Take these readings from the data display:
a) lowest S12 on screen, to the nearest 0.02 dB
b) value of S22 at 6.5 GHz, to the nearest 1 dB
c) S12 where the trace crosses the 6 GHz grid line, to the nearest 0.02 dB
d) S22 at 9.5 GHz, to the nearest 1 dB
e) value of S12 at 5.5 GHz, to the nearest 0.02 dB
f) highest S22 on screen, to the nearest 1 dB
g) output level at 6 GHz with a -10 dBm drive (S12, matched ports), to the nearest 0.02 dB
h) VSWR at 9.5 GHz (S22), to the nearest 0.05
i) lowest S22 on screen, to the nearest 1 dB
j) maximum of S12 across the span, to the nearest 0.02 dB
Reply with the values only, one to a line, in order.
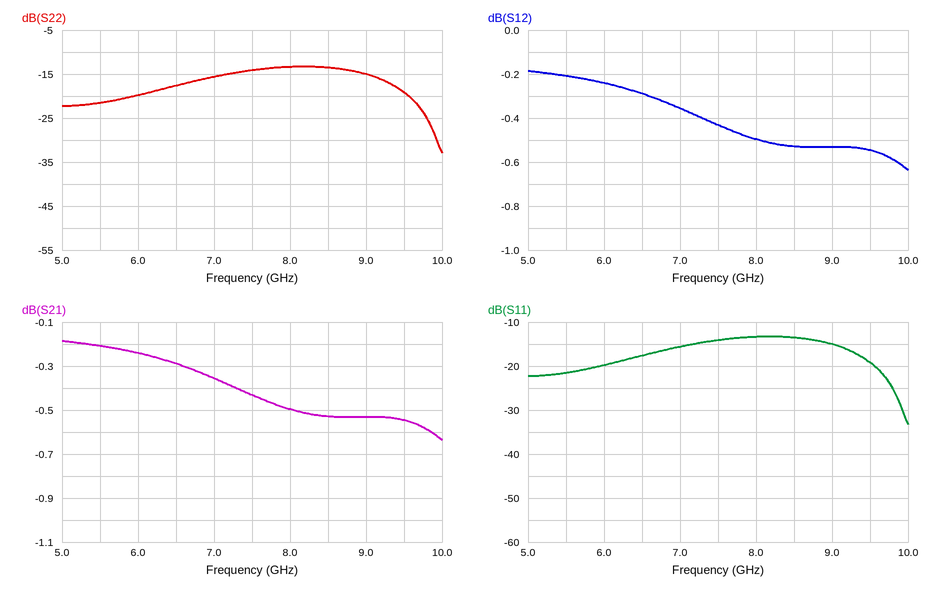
-0.64 dB
-18 dB
-0.24 dB
-19 dB
-0.20 dB
-13 dB
-10.24 dBm
1.25
-33 dB
-0.18 dB
